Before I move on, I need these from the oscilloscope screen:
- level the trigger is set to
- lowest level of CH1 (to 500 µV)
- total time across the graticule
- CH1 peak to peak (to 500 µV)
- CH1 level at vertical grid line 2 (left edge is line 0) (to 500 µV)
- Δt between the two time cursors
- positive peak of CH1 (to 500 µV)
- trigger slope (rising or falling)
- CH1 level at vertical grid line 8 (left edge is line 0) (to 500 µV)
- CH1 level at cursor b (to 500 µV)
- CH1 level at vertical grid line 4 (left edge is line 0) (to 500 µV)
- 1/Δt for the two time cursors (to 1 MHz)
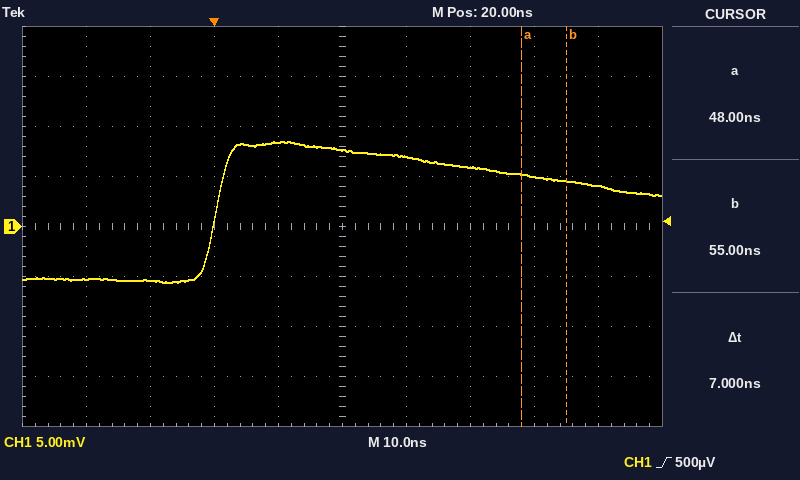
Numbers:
500 µV
-5.5 mV
100 ns
14.0 mV
-5.5 mV
7 ns
8.5 mV
rising
5.0 mV
4.5 mV
8.5 mV
143 MHz
